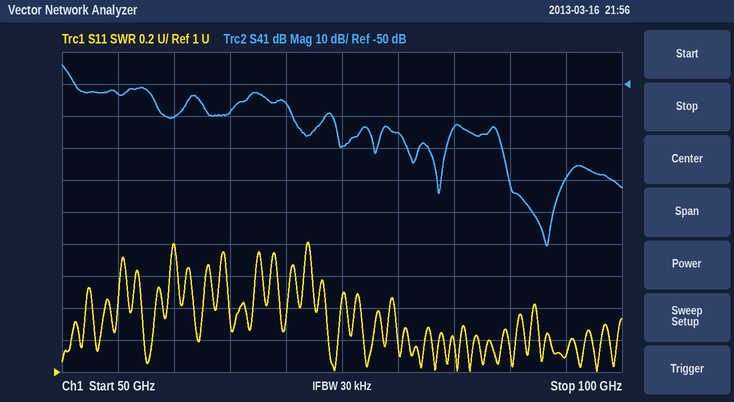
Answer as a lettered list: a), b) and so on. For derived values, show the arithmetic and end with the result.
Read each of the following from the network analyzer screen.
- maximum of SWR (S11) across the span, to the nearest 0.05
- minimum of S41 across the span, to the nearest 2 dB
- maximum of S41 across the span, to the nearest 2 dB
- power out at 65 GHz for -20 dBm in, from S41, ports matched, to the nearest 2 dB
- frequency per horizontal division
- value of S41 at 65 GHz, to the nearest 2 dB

a) 1.80
b) -100 dB
c) -44 dB
d) -20 dBm + (-58 dB) = -78 dBm
e) 5 GHz
f) -58 dB
